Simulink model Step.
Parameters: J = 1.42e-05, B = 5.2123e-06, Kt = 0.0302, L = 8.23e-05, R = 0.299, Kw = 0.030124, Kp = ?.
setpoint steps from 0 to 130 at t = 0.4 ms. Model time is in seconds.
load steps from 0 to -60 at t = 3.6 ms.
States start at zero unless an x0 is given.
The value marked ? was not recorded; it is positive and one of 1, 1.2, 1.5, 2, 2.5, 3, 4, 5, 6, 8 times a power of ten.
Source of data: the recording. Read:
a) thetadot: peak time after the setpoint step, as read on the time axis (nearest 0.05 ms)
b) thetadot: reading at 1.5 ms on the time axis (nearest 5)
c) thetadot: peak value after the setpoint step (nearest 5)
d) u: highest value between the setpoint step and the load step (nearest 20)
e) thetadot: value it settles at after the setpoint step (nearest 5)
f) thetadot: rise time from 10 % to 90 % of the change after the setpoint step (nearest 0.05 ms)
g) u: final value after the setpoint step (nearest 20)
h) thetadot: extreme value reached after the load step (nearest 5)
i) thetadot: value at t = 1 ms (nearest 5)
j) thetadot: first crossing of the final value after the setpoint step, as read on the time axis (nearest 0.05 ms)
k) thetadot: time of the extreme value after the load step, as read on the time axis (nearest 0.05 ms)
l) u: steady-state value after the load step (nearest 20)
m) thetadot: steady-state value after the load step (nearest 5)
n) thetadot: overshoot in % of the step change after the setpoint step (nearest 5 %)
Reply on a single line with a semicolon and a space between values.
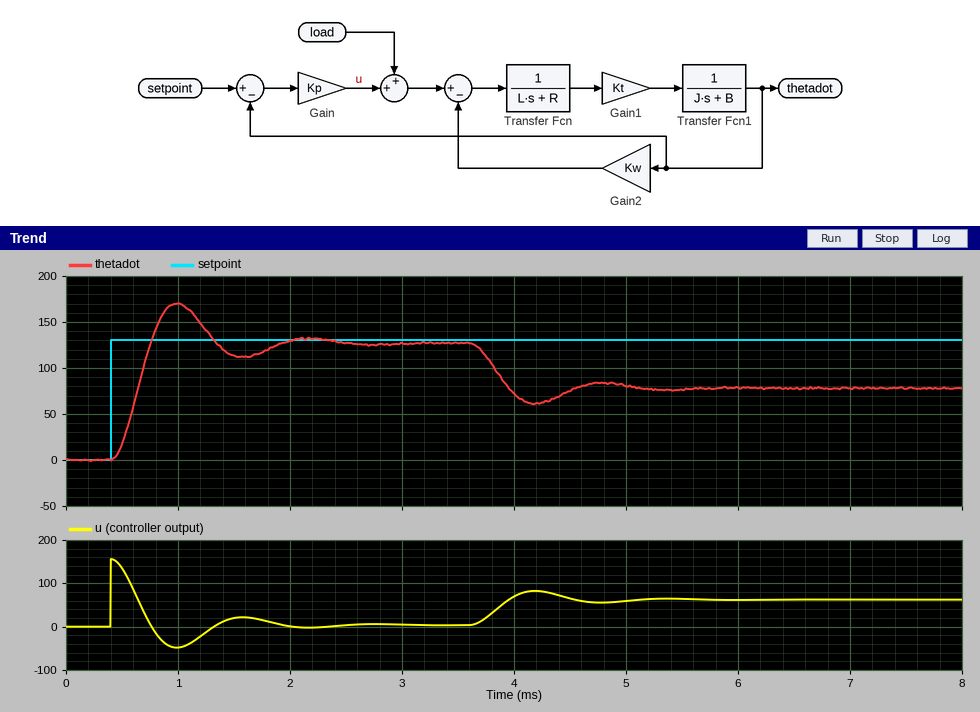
1.00 ms; 115; 170; 160; 125; 0.25 ms; 0; 60; 170; 0.75 ms; 4.20 ms; 60; 80; 35 %
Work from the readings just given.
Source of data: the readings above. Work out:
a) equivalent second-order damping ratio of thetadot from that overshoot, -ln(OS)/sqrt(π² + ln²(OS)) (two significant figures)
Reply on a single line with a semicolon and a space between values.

0.32
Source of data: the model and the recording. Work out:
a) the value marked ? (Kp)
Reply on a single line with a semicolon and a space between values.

1.2
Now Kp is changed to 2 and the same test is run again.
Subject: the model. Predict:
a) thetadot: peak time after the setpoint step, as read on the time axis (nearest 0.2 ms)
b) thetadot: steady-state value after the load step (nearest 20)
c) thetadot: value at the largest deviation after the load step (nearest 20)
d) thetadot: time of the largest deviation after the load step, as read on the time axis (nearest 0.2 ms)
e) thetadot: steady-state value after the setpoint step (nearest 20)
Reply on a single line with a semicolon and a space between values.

0.8 ms; 100; 80; 4.0 ms; 120
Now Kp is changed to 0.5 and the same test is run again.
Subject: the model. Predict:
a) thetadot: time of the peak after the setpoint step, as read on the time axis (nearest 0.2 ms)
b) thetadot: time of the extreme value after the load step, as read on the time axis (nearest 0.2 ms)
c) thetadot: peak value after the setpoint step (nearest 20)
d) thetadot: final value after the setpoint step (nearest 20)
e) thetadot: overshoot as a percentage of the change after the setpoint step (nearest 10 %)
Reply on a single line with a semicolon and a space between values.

1.4 ms; 4.6 ms; 140; 120; 20 %
